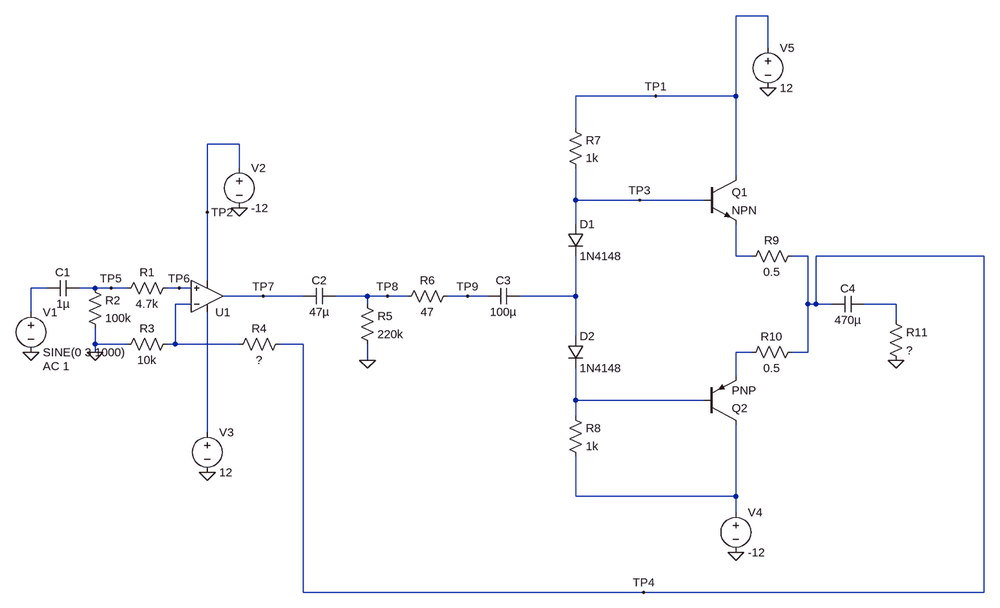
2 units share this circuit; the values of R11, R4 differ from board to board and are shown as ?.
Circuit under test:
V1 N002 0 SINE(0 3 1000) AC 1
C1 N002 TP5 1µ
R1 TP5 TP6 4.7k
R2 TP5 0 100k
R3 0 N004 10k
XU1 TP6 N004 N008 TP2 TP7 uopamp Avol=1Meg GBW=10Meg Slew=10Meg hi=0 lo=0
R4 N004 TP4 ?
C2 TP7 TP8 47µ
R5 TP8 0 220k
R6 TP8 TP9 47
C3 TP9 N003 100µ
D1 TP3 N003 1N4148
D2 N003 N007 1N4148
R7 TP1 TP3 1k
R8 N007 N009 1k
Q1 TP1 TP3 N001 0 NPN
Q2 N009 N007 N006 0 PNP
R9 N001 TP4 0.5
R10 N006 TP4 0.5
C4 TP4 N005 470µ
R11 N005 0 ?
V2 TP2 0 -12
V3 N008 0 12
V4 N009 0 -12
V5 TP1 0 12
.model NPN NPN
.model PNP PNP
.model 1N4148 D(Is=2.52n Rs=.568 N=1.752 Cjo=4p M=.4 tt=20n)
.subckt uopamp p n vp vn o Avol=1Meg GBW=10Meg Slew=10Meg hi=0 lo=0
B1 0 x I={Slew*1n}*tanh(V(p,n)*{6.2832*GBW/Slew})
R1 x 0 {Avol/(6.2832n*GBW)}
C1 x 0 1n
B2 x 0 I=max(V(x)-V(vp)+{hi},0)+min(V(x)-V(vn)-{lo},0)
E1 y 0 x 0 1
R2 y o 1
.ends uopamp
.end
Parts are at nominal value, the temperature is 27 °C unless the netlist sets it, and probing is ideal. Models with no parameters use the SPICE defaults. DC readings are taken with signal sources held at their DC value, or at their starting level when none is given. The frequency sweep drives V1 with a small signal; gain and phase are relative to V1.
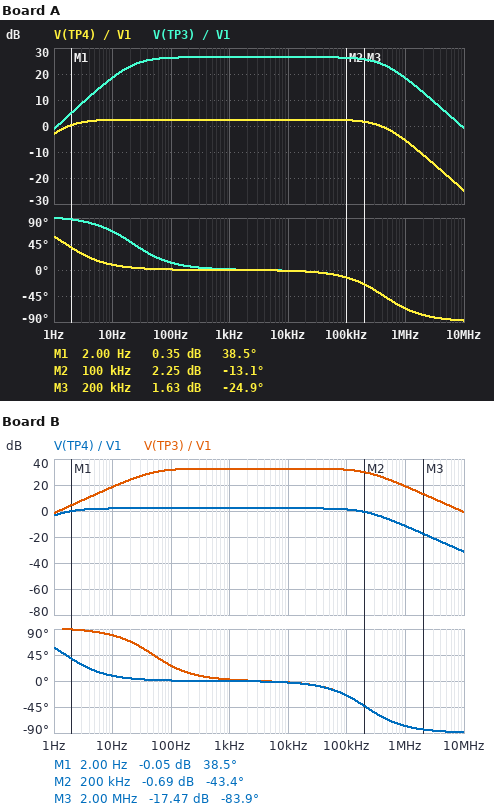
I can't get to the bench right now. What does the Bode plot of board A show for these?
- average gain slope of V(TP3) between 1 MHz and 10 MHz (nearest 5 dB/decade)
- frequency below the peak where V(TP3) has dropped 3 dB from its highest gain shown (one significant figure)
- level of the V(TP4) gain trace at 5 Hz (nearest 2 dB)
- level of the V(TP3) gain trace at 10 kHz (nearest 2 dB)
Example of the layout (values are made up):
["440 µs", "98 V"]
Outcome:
["-20 dB/decade", "20 Hz", "2 dB", "26 dB"]
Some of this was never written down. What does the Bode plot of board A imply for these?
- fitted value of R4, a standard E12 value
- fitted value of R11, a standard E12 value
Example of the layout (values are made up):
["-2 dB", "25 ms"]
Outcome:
["3.3 kΩ", "15 Ω"]
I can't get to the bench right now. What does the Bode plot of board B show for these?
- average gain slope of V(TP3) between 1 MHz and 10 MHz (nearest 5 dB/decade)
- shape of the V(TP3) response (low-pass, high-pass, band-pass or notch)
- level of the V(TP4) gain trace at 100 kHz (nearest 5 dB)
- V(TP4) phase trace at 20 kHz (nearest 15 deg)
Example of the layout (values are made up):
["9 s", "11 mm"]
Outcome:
["-20 dB/decade", "band-pass", "0 dB", "0 deg"]
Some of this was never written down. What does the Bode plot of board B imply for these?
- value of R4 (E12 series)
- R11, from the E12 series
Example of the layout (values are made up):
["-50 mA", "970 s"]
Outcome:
["2.7 kΩ", "6.8 Ω"]
